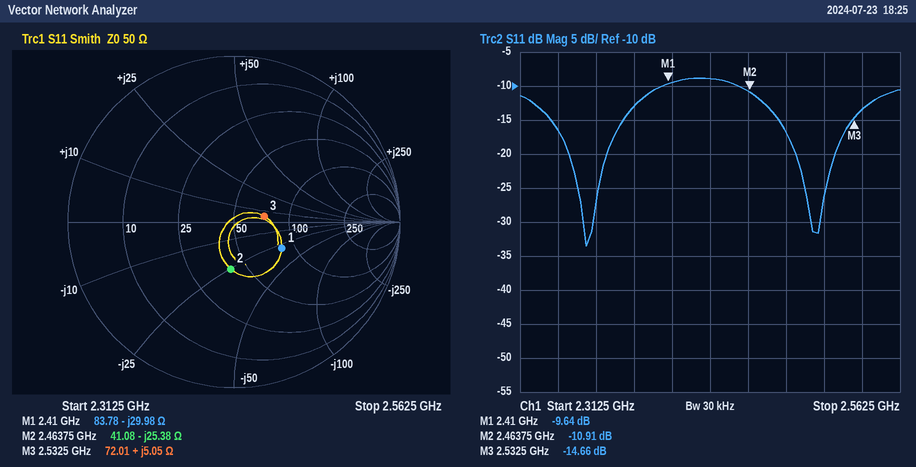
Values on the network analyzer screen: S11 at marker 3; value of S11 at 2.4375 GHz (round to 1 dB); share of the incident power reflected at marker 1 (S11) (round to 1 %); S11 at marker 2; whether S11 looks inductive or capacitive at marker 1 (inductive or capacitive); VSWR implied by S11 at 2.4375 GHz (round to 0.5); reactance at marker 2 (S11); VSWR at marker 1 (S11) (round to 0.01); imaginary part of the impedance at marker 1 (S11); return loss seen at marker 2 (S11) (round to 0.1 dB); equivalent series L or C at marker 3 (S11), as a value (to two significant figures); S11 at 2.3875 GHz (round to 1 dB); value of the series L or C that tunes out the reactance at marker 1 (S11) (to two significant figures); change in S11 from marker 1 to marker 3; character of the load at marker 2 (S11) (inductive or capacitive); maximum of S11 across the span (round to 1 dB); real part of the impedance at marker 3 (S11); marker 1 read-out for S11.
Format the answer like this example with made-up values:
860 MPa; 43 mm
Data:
-14.66 dB; -9 dB; 11 %; -10.91 dB; capacitive; 2.0; -25.38 Ω; 1.98; -29.98 Ω; 10.9 dB; 320 pH; -13 dB; 2.0 nH; -5.02 dB; capacitive; -9 dB; 72.01 Ω; -9.64 dB
